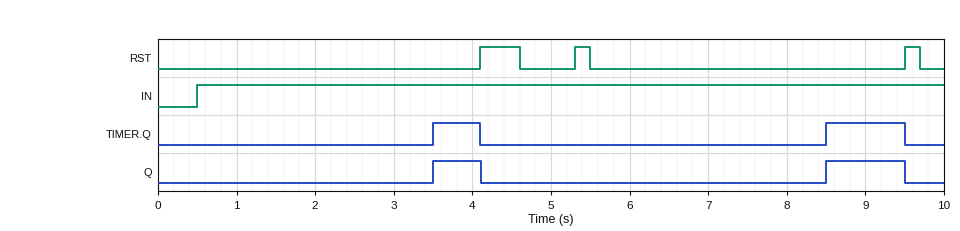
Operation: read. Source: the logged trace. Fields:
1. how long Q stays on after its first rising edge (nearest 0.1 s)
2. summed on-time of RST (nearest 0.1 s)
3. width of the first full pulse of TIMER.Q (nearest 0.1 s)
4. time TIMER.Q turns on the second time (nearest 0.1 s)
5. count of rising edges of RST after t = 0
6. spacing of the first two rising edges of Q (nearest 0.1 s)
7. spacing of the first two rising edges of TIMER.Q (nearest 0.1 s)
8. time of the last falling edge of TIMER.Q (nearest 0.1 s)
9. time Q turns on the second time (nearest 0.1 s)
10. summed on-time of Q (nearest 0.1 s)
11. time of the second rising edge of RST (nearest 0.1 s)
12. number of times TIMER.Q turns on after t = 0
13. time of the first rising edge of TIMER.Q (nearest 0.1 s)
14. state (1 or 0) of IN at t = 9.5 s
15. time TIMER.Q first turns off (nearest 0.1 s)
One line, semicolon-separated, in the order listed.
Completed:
0.6 s; 0.9 s; 0.6 s; 8.5 s; 3; 5.0 s; 5.0 s; 9.5 s; 8.5 s; 1.6 s; 5.3 s; 2; 3.5 s; 1; 4.1 s
